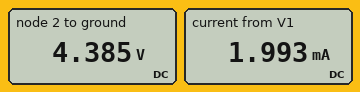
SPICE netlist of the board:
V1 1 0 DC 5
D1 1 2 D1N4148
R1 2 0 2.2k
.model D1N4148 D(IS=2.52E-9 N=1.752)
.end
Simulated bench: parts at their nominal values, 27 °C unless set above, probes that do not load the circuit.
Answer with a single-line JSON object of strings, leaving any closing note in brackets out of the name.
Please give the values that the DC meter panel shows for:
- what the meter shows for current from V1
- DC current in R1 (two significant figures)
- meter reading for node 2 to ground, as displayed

{"what the meter shows for current from V1": "1.993 mA", "DC current in R1": "2.0 mA", "meter reading for node 2 to ground, as displayed": "4.385 V"}
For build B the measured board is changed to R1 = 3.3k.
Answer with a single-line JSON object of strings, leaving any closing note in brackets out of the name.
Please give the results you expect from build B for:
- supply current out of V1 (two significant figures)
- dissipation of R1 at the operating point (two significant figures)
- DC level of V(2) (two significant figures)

{"supply current out of V1": "1.3 mA", "dissipation of R1 at the operating point": "5.9 mW", "DC level of V(2)": "4.4 V"}
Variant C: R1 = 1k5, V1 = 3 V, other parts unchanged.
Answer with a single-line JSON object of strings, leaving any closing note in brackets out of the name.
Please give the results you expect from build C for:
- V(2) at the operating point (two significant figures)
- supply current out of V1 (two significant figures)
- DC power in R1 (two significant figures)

{"V(2) at the operating point": "2.4 V", "supply current out of V1": "1.6 mA", "DC power in R1": "3.8 mW"}
